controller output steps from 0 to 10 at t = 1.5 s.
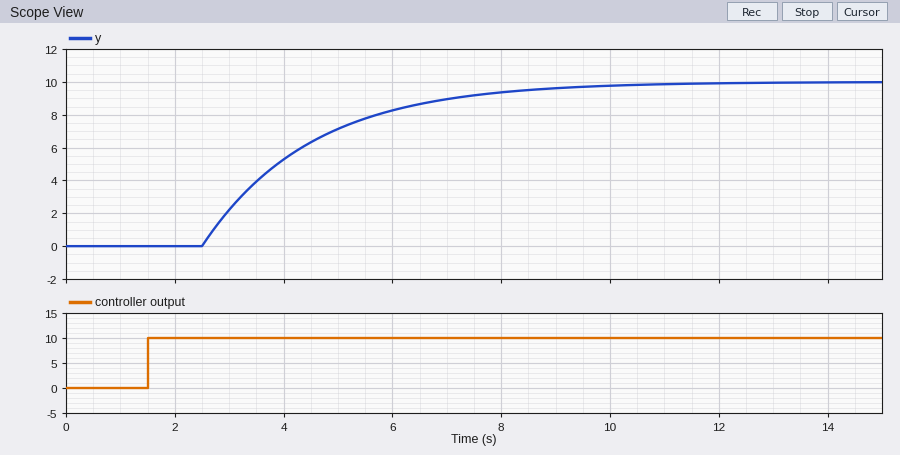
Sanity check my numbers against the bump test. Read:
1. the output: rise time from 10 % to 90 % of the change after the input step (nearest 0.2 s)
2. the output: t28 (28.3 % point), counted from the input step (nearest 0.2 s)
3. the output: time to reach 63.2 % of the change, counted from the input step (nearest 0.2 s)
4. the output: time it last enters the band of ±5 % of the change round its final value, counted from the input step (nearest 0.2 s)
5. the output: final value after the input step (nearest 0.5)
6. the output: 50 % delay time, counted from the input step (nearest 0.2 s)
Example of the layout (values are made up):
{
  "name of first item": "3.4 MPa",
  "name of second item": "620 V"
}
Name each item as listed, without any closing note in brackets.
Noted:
{
  "the output: rise time from 10 % to 90 % of the change after the input step": "4.4 s",
  "the output: t28 (28.3 % point), counted from the input step": "1.6 s",
  "the output: time to reach 63.2 % of the change, counted from the input step": "3.0 s",
  "the output: time it last enters the band of ±5 % of the change round its final value, counted from the input step": "7.0 s",
  "the output: final value after the input step": "10.0",
  "the output: 50 % delay time, counted from the input step": "2.4 s"
}
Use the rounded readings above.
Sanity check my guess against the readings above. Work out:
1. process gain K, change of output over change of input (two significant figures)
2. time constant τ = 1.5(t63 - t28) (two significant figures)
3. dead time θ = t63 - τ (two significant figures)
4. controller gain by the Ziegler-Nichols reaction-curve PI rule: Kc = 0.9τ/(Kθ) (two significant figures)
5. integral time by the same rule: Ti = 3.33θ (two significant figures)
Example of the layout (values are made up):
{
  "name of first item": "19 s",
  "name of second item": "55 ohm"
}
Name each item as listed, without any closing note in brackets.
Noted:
{
  "process gain K, change of output over change of input": "1.0",
  "time constant τ = 1.5(t63 - t28)": "2.1 s",
  "dead time θ = t63 - τ": "0.90 s",
  "controller gain by the Ziegler-Nichols reaction-curve PI rule: Kc = 0.9τ/(Kθ)": "2.1",
  "integral time by the same rule: Ti = 3.33θ": "3.0 s"
}
